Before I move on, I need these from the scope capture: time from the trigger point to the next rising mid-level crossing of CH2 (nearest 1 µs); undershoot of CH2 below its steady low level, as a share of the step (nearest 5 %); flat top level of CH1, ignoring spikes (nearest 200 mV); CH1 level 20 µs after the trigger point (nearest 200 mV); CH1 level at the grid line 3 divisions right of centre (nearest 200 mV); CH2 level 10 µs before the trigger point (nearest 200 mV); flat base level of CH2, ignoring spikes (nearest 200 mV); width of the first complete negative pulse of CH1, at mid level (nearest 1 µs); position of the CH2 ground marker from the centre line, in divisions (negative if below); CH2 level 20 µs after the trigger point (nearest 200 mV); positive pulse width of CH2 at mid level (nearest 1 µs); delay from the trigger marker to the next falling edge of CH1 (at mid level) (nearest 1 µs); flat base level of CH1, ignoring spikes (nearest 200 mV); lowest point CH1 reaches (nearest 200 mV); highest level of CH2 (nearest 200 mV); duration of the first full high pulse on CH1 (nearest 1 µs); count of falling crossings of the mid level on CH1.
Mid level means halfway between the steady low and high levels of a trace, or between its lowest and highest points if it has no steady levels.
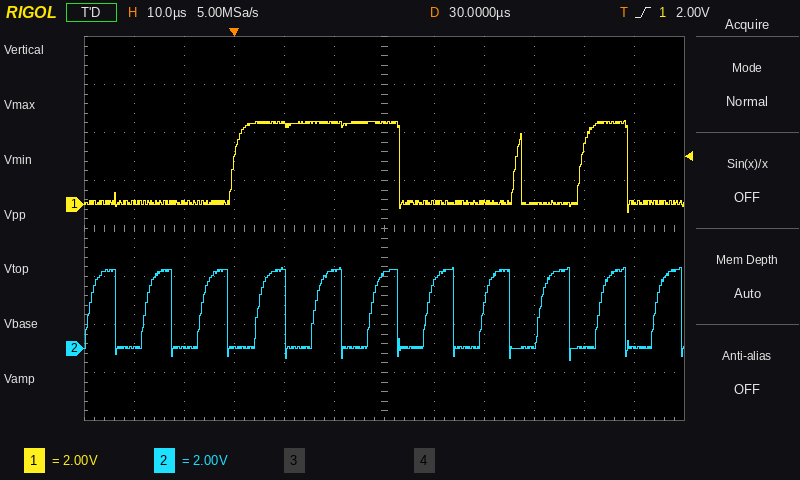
5 µs
15 %
3.4 V
3.4 V
0.0 V
0.0 V
0.0 V
23 µs
-2.5 div
3.2 V
5 µs
33 µs
0.0 V
-400 mV
3.4 V
33 µs
3
